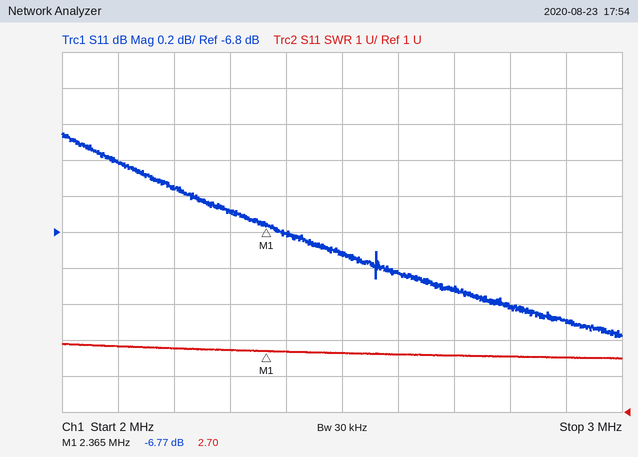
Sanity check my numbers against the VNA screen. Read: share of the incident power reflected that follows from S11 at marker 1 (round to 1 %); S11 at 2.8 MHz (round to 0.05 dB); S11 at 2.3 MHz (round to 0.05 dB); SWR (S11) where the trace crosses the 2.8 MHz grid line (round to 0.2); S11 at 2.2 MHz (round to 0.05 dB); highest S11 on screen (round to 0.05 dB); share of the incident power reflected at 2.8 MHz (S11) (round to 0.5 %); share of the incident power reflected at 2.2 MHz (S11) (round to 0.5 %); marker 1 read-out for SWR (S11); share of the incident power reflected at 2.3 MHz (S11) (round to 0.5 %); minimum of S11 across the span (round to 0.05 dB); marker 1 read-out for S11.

21 %
-7.20 dB
-6.70 dB
2.6
-6.55 dB
-6.25 dB
19.0 %
22.0 %
2.70
21.5 %
-7.40 dB
-6.77 dB
